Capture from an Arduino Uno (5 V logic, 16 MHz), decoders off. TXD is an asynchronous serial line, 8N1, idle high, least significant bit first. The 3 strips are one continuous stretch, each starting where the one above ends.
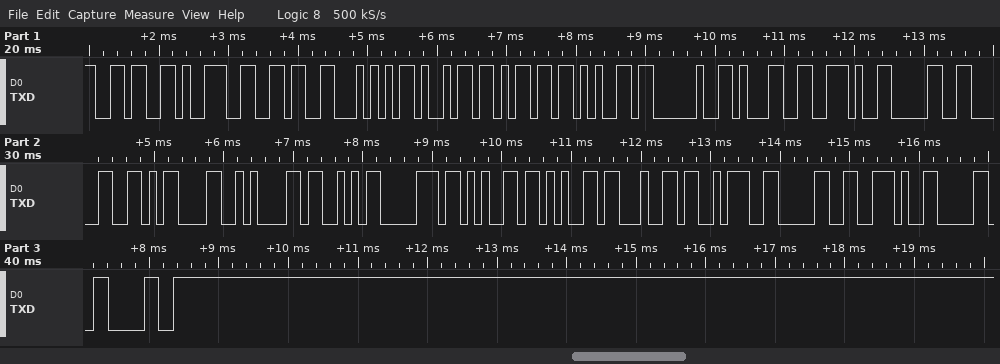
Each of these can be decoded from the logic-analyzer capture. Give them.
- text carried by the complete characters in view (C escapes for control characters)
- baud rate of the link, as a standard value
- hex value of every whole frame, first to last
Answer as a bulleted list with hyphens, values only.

- "696Time 1.00\r\nSpeed:0.00"
- 9600 baud
- 36 39 36 54 69 6D 65 20 31 2E 30 30 0D 0A 53 70 65 65 64 3A 30 2E 30 30
